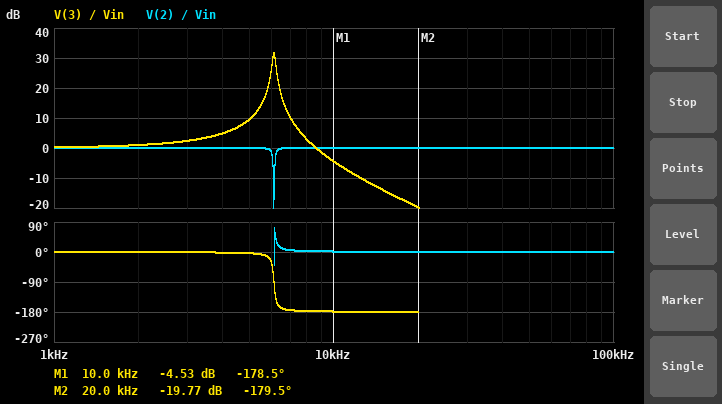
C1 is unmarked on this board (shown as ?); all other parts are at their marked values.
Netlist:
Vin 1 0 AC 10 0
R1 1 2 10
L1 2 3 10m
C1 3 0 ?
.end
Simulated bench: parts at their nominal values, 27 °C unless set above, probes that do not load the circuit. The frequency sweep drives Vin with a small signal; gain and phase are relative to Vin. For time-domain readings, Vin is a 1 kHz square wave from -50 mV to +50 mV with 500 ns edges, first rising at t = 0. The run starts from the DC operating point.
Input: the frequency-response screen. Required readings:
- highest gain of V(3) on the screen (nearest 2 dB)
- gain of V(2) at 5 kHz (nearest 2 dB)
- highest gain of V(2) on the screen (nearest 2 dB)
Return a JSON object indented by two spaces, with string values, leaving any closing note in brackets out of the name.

{
  "highest gain of V(3) on the screen": "32 dB",
  "gain of V(2) at 5 kHz": "0 dB",
  "highest gain of V(2) on the screen": "0 dB"
}
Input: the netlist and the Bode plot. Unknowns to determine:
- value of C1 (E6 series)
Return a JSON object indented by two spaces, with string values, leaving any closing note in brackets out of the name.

{
  "value of C1": "68 nF"
}
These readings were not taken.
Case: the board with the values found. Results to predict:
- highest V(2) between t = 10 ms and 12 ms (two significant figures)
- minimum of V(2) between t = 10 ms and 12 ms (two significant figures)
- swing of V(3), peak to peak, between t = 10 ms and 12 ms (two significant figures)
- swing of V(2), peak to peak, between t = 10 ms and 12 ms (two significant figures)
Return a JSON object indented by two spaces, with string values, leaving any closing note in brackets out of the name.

{
  "highest V(2) between t = 10 ms and 12 ms": "51 mV",
  "minimum of V(2) between t = 10 ms and 12 ms": "-51 mV",
  "swing of V(3), peak to peak, between t = 10 ms and 12 ms": "210 mV",
  "swing of V(2), peak to peak, between t = 10 ms and 12 ms": "100 mV"
}
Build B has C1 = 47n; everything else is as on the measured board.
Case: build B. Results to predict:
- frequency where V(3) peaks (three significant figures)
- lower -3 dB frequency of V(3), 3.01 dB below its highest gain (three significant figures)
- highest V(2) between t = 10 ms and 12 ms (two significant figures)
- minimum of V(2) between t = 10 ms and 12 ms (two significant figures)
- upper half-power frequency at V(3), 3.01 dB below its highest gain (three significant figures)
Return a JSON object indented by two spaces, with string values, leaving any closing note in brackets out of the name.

{
  "frequency where V(3) peaks": "7.34 kHz",
  "lower -3 dB frequency of V(3), 3.01 dB below its highest gain": "7.26 kHz",
  "highest V(2) between t = 10 ms and 12 ms": "52 mV",
  "minimum of V(2) between t = 10 ms and 12 ms": "-52 mV",
  "upper half-power frequency at V(3), 3.01 dB below its highest gain": "7.42 kHz"
}
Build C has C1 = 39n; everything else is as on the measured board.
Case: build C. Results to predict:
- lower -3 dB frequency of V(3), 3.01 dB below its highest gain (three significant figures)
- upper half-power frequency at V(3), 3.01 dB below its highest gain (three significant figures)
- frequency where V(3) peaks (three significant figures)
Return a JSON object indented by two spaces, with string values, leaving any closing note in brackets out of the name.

{
  "lower -3 dB frequency of V(3), 3.01 dB below its highest gain": "7.98 kHz",
  "upper half-power frequency at V(3), 3.01 dB below its highest gain": "8.14 kHz",
  "frequency where V(3) peaks": "8.06 kHz"
}
